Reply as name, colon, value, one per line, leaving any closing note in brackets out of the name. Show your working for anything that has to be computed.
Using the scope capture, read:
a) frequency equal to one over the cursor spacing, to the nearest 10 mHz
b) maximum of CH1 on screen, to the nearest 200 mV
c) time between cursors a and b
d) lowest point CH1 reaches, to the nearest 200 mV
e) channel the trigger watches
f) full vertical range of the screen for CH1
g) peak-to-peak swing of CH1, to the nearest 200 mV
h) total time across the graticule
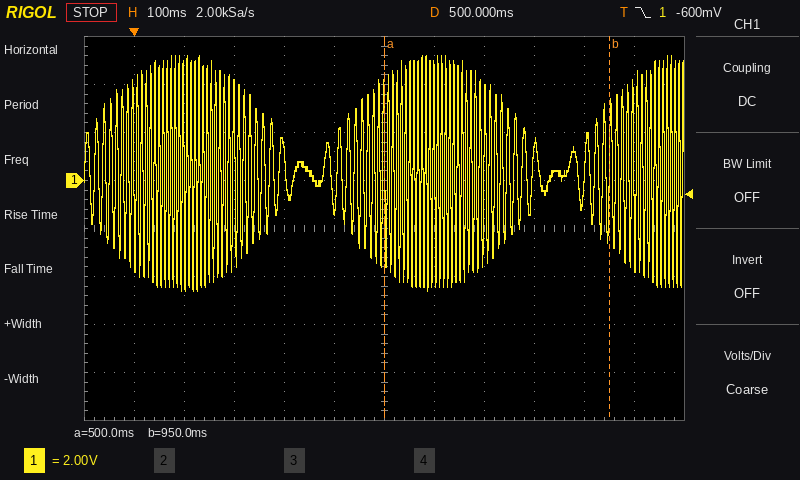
frequency equal to one over the cursor spacing, to the nearest 10 mHz: 1 / 450 ms ≈ 2.22 Hz
maximum of CH1 on screen, to the nearest 200 mV: 5.2 V
time between cursors a and b: 950 ms − (500 ms) = 450 ms
lowest point CH1 reaches, to the nearest 200 mV: -4.6 V
channel the trigger watches: CH1
full vertical range of the screen for CH1: 16 V
peak-to-peak swing of CH1, to the nearest 200 mV: 5.2 V − (-4.6 V) = 9.8 V
total time across the graticule: 1.2 s
